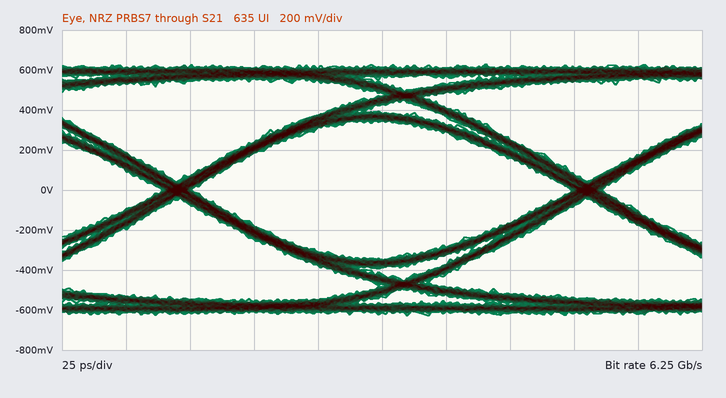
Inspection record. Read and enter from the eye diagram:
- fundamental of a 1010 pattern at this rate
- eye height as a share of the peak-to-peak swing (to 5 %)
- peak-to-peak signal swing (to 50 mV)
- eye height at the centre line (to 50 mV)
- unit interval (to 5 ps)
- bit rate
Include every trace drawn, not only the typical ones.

3.125 GHz
55 %
1.25 V
700 mV
160 ps
6.25 Gb/s
